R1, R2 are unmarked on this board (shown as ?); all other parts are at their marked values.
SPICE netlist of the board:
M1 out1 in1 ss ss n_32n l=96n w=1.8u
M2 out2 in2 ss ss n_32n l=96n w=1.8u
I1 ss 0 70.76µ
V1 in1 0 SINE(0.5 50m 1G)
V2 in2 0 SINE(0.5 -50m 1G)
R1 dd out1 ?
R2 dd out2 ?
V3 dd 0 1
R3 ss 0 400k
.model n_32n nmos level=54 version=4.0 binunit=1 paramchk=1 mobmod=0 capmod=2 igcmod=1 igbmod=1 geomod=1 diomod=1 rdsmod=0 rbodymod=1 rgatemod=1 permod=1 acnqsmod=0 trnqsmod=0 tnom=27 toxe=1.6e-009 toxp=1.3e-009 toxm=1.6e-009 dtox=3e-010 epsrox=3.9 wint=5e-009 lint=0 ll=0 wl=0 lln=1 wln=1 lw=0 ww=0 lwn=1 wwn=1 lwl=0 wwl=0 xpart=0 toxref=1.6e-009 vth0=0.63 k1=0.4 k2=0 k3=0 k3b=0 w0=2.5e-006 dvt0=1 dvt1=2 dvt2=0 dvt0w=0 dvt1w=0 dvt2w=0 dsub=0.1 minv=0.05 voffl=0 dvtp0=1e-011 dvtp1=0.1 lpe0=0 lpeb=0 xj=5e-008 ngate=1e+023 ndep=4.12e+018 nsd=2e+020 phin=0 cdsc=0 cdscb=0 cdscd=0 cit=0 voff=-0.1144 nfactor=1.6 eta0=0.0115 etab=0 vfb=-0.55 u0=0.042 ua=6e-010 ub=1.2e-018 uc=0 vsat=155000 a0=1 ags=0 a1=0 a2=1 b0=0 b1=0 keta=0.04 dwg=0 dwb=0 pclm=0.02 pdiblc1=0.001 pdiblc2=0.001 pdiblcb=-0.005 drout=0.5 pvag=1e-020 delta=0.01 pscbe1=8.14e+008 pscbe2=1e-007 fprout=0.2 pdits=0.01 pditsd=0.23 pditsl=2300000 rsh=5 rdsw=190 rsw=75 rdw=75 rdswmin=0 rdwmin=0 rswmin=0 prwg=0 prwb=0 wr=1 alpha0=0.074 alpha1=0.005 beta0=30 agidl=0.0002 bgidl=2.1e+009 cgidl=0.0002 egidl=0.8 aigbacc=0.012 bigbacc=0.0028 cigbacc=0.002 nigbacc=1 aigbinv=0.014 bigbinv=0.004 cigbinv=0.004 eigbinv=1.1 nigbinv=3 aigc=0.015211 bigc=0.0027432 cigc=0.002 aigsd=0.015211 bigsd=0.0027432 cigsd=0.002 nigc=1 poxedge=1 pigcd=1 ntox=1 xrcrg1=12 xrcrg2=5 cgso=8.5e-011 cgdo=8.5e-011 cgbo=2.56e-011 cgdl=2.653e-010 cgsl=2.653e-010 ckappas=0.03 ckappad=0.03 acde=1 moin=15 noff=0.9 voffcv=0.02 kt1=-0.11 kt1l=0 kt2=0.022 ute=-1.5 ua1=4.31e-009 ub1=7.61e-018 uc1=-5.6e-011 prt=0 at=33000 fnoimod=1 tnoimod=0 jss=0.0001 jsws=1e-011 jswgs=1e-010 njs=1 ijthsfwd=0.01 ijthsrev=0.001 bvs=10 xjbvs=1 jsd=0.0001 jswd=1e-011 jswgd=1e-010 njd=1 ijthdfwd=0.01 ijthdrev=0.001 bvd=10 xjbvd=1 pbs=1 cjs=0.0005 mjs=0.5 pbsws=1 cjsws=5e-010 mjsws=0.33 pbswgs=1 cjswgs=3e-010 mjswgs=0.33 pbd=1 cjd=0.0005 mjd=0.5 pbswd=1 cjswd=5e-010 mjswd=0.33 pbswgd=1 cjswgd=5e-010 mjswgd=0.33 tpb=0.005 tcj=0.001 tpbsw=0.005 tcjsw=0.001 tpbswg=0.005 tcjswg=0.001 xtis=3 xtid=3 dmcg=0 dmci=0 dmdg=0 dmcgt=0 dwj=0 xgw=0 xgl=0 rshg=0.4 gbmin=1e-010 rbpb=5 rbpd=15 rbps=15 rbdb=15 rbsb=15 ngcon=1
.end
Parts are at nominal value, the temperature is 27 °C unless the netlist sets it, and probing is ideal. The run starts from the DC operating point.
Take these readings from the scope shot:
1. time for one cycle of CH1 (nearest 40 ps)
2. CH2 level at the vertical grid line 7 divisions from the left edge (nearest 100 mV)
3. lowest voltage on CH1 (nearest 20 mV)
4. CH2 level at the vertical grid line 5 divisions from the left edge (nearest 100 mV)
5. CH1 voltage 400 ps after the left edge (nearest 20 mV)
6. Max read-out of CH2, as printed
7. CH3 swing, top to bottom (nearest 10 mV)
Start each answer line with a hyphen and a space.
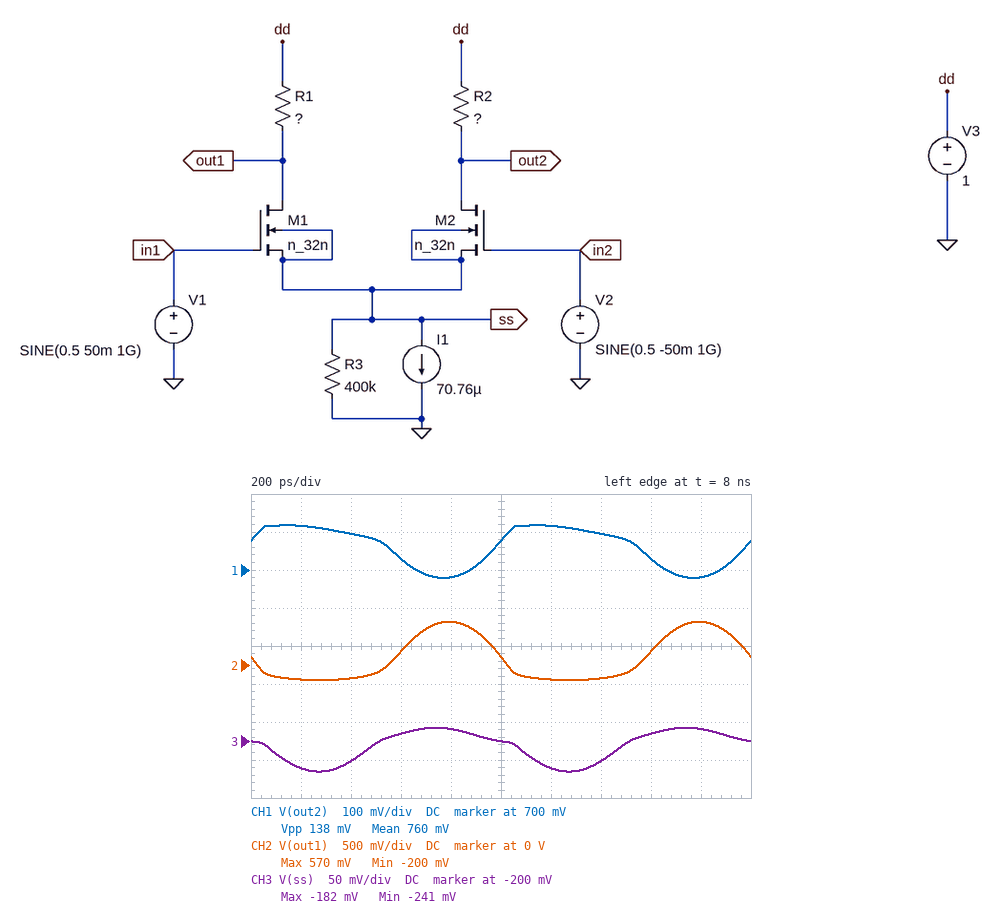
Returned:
- 1.00 ns
- -200 mV
- 680 mV
- 100 mV
- 800 mV
- 570 mV
- 60 mV
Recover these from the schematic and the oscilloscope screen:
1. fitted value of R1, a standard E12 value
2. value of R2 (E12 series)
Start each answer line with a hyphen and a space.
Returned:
- 33 kΩ
- 5.6 kΩ
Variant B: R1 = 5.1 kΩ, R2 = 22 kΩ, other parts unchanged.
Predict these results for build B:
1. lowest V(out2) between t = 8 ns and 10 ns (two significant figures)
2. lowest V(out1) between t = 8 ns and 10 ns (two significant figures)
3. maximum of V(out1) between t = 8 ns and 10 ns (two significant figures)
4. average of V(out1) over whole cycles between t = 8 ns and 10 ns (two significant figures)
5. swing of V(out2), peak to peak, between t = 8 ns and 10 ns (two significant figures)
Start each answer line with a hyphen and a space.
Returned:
- -110 mV
- 710 mV
- 900 mV
- 810 mV
- 830 mV
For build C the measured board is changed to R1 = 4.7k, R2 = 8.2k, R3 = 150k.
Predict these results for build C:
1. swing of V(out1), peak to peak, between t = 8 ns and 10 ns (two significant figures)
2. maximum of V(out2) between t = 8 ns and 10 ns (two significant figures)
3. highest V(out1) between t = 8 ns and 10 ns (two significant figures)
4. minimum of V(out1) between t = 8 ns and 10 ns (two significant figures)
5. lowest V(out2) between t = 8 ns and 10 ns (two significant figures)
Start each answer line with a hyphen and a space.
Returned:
- 200 mV
- 890 mV
- 940 mV
- 730 mV
- 540 mV
